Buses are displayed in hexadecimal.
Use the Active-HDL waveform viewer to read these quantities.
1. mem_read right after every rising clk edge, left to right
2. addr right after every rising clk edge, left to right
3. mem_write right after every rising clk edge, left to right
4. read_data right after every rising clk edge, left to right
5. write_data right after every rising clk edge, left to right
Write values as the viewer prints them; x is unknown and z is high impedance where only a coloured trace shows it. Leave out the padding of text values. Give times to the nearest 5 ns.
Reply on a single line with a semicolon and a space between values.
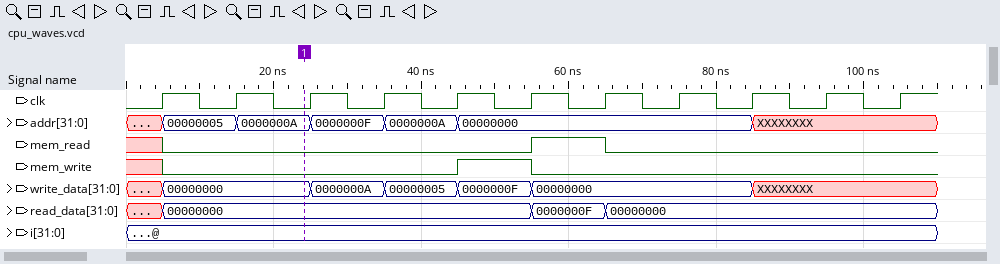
0 0 0 0 0 1 0 0 0 0 0; 00000005, 0000000A, 0000000F, 0000000A, 00000000, 00000000, 00000000, 00000000, XXXXXXXX, XXXXXXXX, XXXXXXXX; 0 0 0 0 1 0 0 0 0 0 0; 00000000, 00000000, 00000000, 00000000, 00000000, 0000000F, 00000000, 00000000, 00000000, 00000000, 00000000; 00000000, 00000000, 0000000A, 00000005, 0000000F, 00000000, 00000000, 00000000, XXXXXXXX, XXXXXXXX, XXXXXXXX
